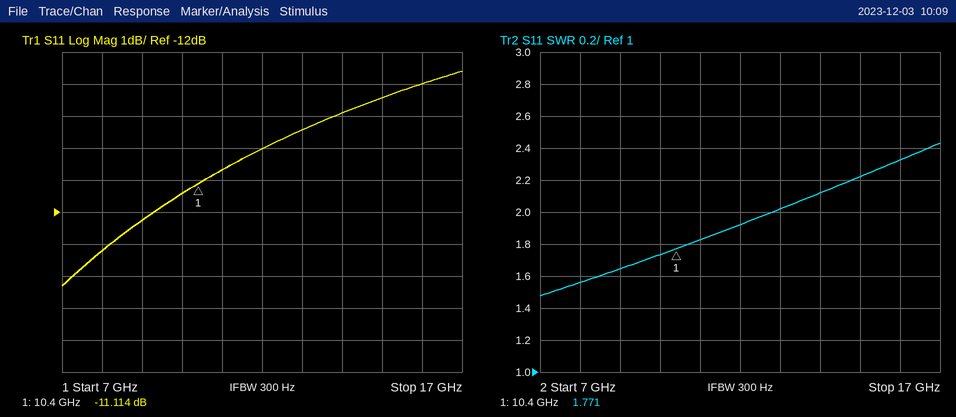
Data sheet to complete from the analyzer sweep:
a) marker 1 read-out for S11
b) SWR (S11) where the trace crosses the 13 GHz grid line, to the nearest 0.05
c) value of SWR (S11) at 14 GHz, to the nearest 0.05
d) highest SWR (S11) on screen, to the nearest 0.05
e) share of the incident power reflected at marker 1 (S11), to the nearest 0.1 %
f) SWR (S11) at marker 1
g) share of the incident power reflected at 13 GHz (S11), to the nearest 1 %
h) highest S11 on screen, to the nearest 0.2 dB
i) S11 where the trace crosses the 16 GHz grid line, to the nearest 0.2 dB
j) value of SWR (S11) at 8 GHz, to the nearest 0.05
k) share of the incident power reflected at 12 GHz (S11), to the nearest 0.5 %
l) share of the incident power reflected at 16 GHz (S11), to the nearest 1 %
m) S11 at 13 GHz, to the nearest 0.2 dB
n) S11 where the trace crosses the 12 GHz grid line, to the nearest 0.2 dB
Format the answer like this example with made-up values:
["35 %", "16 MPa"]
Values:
["-11.114 dB", "2.00", "2.10", "2.45", "7.7 %", "1.771", "11 %", "-7.6 dB", "-8.0 dB", "1.55", "10.0 %", "16 %", "-9.4 dB", "-10.0 dB"]
